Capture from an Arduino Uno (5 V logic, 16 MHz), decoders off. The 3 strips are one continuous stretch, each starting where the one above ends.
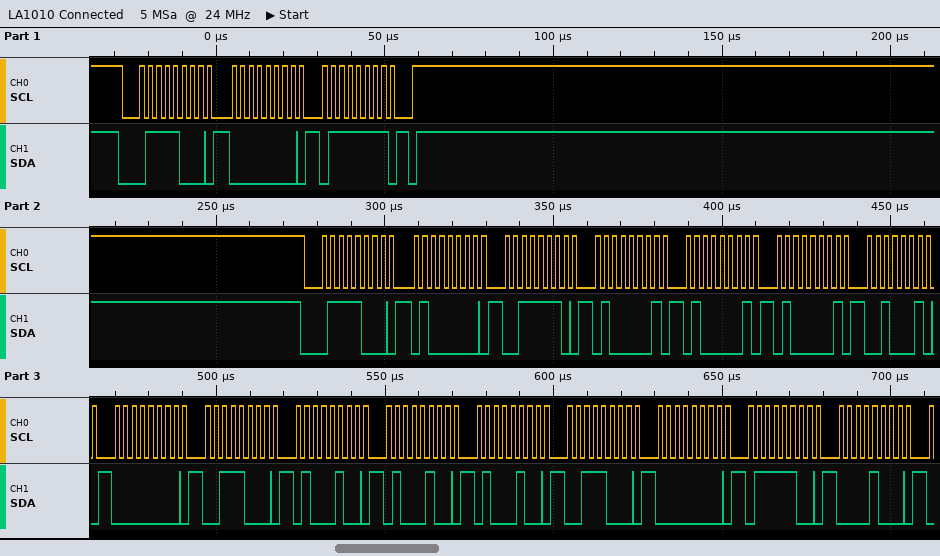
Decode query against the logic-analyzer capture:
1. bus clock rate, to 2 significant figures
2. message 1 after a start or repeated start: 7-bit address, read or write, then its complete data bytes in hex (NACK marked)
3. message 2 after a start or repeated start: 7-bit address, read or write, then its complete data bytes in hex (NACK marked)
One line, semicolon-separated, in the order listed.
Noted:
400 kHz; 0x3C write: 00 7F; 0x3C write: 40 3E 41 41 41 22 00 38 44 44 44 38 00 7C 08
